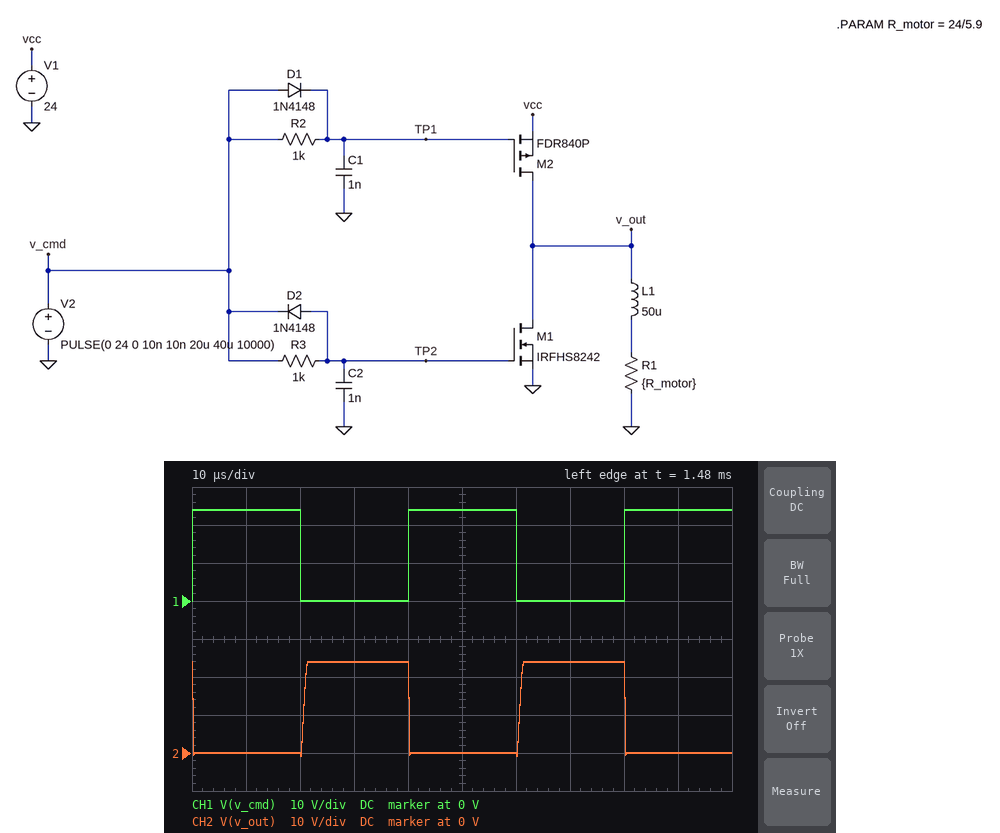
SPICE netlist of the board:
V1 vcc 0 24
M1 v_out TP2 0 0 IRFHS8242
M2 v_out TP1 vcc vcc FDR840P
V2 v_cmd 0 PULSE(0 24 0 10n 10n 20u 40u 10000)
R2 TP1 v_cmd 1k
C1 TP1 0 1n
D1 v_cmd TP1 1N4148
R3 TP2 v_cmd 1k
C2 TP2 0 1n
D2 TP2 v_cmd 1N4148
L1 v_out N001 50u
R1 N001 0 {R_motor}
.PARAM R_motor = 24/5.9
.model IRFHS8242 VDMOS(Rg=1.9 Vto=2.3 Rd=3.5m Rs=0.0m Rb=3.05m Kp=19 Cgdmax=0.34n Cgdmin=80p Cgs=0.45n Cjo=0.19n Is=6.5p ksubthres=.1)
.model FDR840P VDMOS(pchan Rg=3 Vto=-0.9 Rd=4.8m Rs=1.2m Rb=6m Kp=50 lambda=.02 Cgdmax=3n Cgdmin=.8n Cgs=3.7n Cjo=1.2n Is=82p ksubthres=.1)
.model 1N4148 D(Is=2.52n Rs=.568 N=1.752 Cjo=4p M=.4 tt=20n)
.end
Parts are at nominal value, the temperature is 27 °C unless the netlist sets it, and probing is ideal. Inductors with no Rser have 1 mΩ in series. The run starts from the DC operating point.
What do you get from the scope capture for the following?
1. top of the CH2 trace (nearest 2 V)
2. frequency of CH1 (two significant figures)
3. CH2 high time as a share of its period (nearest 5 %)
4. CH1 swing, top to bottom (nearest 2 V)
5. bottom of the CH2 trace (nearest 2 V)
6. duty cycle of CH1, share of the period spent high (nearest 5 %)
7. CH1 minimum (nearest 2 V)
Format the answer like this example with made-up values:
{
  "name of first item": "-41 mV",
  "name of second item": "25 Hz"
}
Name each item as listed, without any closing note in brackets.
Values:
{
  "top of the CH2 trace": "24 V",
  "frequency of CH1": "25 kHz",
  "CH2 high time as a share of its period": "50 %",
  "CH1 swing, top to bottom": "24 V",
  "bottom of the CH2 trace": "0 V",
  "duty cycle of CH1, share of the period spent high": "50 %",
  "CH1 minimum": "0 V"
}
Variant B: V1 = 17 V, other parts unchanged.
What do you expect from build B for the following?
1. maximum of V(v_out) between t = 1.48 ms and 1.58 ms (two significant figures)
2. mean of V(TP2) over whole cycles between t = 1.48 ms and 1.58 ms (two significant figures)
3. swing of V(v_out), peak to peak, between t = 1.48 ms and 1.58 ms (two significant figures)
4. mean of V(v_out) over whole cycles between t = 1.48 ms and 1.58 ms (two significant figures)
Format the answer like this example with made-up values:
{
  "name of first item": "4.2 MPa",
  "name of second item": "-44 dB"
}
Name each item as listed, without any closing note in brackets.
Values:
{
  "maximum of V(v_out) between t = 1.48 ms and 1.58 ms": "17 V",
  "mean of V(TP2) over whole cycles between t = 1.48 ms and 1.58 ms": "11 V",
  "swing of V(v_out), peak to peak, between t = 1.48 ms and 1.58 ms": "18 V",
  "mean of V(v_out) over whole cycles between t = 1.48 ms and 1.58 ms": "7.3 V"
}
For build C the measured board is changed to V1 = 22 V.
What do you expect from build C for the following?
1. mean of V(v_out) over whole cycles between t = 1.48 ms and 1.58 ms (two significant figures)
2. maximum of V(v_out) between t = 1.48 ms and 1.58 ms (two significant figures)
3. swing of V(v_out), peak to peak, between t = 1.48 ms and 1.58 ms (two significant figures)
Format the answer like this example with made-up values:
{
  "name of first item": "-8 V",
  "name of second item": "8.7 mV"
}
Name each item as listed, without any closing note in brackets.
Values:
{
  "mean of V(v_out) over whole cycles between t = 1.48 ms and 1.58 ms": "10 V",
  "maximum of V(v_out) between t = 1.48 ms and 1.58 ms": "22 V",
  "swing of V(v_out), peak to peak, between t = 1.48 ms and 1.58 ms": "23 V"
}
